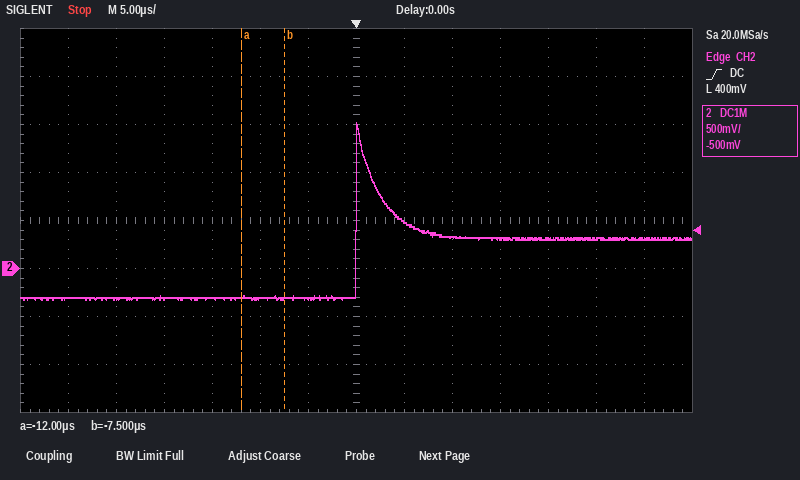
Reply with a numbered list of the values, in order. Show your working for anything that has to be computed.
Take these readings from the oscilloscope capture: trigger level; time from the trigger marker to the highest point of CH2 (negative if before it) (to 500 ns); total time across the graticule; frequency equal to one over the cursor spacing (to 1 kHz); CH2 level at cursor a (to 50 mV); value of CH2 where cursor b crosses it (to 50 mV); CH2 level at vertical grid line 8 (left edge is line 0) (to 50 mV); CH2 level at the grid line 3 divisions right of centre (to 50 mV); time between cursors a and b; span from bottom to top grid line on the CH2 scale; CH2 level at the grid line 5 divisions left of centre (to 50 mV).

1. 400 mV
2. 0.0 µs
3. 70 µs
4. 1 / 4.5 µs ≈ 222 kHz
5. -300 mV
6. -300 mV
7. 500 mV
8. 300 mV
9. -7.5 µs − (-12 µs) = 4.5 µs
10. 4 V
11. -300 mV
